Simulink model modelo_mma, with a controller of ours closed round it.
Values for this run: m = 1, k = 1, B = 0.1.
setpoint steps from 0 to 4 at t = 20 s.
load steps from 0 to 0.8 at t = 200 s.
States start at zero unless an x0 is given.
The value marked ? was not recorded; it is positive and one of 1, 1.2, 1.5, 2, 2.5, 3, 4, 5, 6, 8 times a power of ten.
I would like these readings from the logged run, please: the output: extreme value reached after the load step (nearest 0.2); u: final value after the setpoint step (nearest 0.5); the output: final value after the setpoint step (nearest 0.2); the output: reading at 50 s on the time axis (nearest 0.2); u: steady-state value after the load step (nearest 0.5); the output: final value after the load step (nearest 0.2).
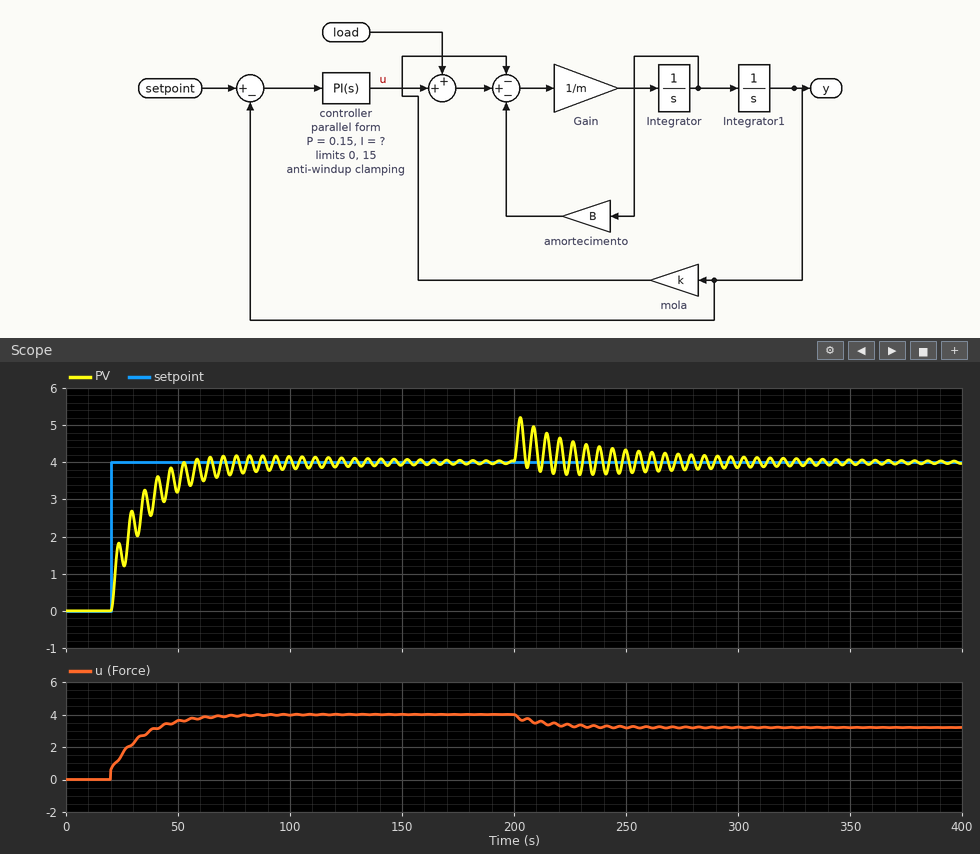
5.2
4.0
4.0
3.2
3.0
4.0
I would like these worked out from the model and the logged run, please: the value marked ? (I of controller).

0.08
